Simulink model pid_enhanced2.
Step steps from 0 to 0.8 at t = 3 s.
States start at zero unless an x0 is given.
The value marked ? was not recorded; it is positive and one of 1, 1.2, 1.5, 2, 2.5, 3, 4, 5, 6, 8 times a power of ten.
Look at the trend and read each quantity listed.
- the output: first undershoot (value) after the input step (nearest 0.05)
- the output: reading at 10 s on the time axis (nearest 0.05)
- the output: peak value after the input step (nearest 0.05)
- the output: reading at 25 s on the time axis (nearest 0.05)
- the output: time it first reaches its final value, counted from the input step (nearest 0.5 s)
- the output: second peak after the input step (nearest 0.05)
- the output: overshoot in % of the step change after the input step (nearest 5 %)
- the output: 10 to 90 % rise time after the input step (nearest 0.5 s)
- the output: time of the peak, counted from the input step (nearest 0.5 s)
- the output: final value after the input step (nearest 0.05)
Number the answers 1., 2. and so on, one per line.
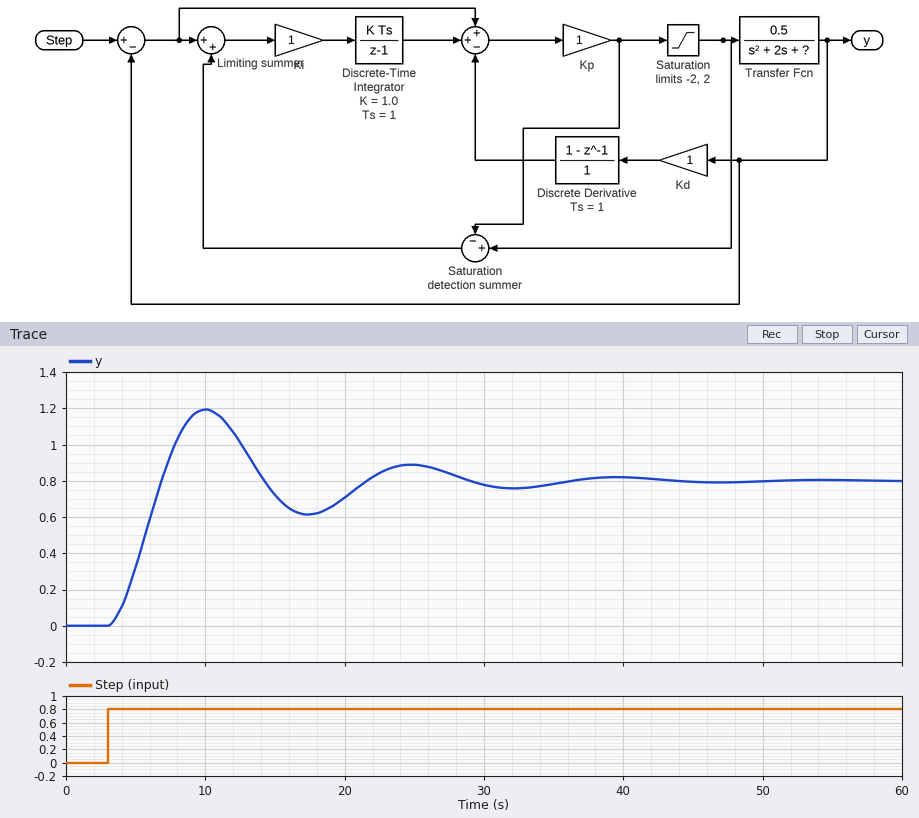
1. 0.60
2. 1.20
3. 1.20
4. 0.90
5. 4.0 s
6. 0.90
7. 50 %
8. 2.5 s
9. 7.0 s
10. 0.80
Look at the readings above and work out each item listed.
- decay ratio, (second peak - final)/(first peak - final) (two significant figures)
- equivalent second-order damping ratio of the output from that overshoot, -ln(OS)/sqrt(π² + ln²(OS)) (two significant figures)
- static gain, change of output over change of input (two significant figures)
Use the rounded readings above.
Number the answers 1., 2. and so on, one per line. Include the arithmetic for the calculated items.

1. (0.9 - 0.8) / (1.2 - 0.8) = 0.25
2. ln(0.5) = -0.693; 0.693 / sqrt(9.870 + 0.480) = 0.22
3. (0.8 - 0) / (0.8 - 0) = 1.0
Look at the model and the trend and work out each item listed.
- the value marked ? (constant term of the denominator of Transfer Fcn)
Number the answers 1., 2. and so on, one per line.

1. 0.6
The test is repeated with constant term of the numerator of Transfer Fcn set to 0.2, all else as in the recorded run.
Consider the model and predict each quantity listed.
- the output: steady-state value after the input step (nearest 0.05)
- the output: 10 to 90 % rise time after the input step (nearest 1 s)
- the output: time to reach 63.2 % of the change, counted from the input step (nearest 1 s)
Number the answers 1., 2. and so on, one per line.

1. 0.65
2. 7 s
3. 4 s
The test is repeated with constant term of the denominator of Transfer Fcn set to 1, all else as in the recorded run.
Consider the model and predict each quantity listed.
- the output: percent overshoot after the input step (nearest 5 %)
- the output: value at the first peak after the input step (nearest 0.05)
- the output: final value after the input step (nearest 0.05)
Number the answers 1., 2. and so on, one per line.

1. 20 %
2. 0.95
3. 0.80
